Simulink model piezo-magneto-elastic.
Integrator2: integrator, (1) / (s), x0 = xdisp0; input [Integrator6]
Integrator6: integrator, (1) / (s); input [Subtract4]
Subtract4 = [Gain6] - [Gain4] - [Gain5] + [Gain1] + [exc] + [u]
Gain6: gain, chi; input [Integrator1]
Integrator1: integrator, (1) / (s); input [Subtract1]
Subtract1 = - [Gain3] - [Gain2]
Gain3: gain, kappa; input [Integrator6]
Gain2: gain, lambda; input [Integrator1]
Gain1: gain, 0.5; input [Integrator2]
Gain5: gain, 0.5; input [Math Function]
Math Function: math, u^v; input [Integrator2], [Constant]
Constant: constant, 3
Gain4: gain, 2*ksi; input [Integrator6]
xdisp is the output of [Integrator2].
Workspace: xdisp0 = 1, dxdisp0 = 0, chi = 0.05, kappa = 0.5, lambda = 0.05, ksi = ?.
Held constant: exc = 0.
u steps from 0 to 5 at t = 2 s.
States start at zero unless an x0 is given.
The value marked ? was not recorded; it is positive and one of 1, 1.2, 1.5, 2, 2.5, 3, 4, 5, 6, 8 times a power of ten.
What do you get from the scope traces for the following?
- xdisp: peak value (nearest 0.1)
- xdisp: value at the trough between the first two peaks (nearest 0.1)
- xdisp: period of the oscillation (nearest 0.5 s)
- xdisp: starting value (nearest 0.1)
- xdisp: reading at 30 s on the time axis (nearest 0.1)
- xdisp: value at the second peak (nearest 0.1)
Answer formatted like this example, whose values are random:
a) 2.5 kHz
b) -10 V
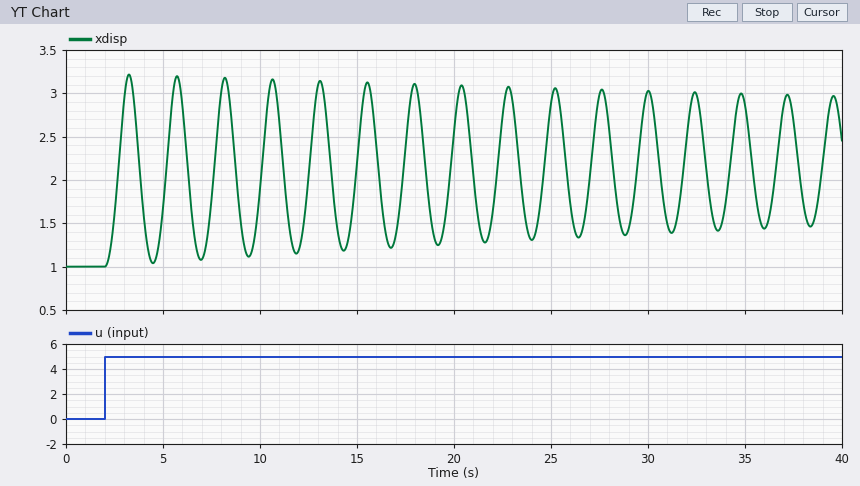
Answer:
a) 3.2
b) 1.0
c) 2.5 s
d) 1.0
e) 3.0
f) 3.2
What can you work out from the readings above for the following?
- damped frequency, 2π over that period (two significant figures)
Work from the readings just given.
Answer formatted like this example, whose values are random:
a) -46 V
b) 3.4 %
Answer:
a) 2.5 rad/s
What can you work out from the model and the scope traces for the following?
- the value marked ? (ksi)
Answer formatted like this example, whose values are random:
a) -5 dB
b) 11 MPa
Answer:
a) 0.01
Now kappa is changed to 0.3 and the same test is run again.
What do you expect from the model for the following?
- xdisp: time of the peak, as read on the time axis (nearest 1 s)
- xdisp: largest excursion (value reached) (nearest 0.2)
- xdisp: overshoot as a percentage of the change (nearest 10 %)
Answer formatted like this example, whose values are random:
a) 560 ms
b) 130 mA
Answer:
a) 3 s
b) 3.2
c) 80 %
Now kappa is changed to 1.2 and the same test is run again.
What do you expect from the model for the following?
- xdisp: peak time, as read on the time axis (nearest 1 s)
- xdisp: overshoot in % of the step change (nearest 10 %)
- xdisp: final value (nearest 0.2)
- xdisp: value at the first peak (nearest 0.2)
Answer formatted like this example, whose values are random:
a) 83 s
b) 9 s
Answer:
a) 3 s
b) 80 %
c) 2.2
d) 3.2
